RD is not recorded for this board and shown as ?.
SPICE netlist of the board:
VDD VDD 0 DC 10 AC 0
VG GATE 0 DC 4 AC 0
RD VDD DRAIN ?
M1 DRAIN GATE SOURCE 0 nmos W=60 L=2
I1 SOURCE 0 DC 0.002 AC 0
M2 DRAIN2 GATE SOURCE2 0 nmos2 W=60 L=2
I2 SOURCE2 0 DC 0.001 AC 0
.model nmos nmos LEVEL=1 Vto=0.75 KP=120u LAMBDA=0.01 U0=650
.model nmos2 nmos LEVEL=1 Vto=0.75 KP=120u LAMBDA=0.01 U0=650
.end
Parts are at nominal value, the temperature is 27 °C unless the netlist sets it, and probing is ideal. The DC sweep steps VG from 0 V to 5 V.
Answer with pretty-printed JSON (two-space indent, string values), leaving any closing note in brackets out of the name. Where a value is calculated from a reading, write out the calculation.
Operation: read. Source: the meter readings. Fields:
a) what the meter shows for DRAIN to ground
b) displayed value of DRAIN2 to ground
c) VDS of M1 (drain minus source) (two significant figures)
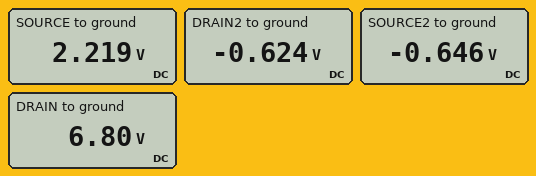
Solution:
{
  "what the meter shows for DRAIN to ground": "6.80 V",
  "displayed value of DRAIN2 to ground": "-0.624 V",
  "VDS of M1 (drain minus source)": "6.8 V - 2.219 V = 4.6 V"
}
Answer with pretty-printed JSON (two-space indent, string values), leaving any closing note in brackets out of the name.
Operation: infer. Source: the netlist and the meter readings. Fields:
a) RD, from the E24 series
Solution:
{
  "RD, from the E24 series": "1.6 kΩ"
}
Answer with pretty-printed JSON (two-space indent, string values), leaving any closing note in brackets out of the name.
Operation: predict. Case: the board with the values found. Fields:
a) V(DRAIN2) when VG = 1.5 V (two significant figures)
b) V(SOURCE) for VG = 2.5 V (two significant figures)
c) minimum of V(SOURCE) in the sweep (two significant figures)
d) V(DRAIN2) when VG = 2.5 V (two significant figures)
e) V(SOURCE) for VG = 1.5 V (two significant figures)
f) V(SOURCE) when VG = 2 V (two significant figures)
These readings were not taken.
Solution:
{
  "V(DRAIN2) when VG = 1.5 V": "-610 mV",
  "V(SOURCE) for VG = 2.5 V": "730 mV",
  "minimum of V(SOURCE) in the sweep": "-670 mV",
  "V(DRAIN2) when VG = 2.5 V": "-620 mV",
  "V(SOURCE) for VG = 1.5 V": "-270 mV",
  "V(SOURCE) when VG = 2 V": "230 mV"
}
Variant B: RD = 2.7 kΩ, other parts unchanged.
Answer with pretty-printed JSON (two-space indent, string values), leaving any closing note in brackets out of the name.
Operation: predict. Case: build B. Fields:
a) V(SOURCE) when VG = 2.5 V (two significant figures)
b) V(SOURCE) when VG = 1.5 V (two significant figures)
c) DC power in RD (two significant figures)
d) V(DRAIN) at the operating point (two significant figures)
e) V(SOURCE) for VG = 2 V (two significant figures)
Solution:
{
  "V(SOURCE) when VG = 2.5 V": "720 mV",
  "V(SOURCE) when VG = 1.5 V": "-280 mV",
  "DC power in RD": "11 mW",
  "V(DRAIN) at the operating point": "4.6 V",
  "V(SOURCE) for VG = 2 V": "220 mV"
}
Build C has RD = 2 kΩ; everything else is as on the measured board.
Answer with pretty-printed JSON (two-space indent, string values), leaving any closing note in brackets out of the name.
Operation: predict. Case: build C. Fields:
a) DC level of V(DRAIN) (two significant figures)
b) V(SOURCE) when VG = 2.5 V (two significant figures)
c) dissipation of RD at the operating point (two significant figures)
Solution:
{
  "DC level of V(DRAIN)": "6.0 V",
  "V(SOURCE) when VG = 2.5 V": "720 mV",
  "dissipation of RD at the operating point": "8.0 mW"
}
